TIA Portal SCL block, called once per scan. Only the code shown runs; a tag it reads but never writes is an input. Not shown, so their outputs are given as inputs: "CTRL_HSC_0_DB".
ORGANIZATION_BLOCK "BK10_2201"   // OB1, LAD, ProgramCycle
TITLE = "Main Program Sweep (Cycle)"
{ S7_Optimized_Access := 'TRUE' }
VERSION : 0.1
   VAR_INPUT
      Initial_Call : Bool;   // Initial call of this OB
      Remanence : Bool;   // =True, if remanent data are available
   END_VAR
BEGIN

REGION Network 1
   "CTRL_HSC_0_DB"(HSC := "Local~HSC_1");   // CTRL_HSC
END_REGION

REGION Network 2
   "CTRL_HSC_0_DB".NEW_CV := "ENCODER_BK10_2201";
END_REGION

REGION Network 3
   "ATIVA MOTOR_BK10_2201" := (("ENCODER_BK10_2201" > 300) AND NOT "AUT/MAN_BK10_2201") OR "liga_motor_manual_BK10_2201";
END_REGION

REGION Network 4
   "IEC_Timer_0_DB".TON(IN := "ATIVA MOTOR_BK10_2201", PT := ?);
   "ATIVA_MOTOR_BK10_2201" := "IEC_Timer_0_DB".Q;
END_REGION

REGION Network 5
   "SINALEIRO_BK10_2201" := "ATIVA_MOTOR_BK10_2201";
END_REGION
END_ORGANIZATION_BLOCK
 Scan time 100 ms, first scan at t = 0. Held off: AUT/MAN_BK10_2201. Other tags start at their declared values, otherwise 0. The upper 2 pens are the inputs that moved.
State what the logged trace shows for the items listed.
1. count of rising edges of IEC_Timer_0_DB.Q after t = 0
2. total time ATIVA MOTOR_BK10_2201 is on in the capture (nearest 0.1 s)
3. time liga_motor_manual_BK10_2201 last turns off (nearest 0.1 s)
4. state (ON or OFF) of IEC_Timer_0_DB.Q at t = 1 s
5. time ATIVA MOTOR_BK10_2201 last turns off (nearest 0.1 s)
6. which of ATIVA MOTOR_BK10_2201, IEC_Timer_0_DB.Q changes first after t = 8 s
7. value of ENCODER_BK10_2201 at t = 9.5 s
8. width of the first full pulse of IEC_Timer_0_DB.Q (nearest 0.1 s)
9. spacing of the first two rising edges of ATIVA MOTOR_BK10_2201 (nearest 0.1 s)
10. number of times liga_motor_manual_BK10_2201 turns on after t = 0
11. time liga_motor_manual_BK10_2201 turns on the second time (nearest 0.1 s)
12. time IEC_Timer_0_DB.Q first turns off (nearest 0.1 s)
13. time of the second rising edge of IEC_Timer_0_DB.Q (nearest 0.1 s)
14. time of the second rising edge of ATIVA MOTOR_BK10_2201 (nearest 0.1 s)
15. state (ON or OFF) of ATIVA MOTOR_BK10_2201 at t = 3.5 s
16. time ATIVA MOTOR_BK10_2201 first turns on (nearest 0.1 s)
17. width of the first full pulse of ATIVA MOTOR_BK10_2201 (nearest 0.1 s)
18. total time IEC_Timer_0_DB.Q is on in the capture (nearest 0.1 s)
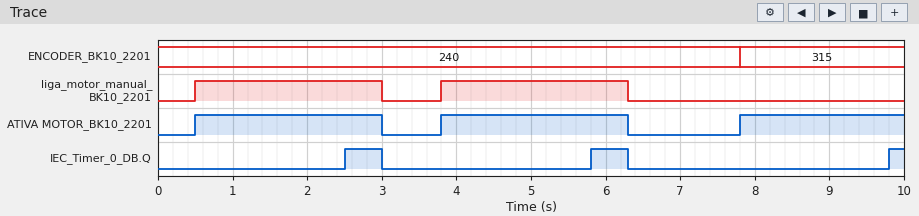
3
7.2 s
6.3 s
OFF
6.3 s
IEC_Timer_0_DB.Q
315
0.5 s
3.3 s
2
3.8 s
3.0 s
5.8 s
3.8 s
OFF
0.5 s
2.5 s
1.2 s
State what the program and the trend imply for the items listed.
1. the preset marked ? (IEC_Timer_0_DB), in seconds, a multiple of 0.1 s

2.0 s
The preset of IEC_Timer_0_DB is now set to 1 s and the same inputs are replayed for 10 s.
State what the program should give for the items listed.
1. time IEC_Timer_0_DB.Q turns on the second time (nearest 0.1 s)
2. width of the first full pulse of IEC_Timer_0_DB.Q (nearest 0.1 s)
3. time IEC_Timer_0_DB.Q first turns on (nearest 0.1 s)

4.8 s
1.5 s
1.5 s
